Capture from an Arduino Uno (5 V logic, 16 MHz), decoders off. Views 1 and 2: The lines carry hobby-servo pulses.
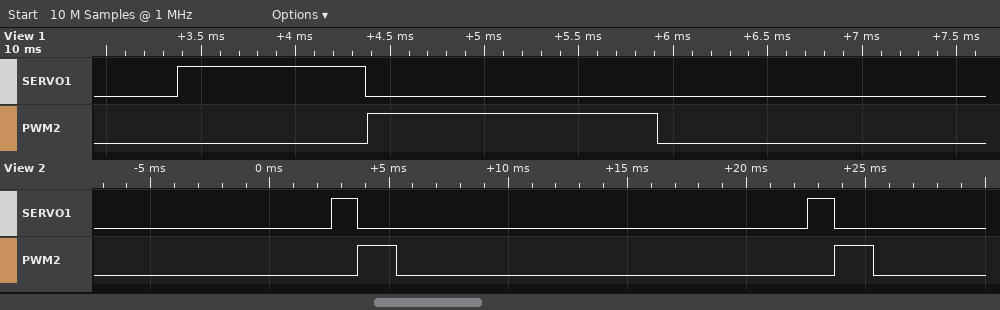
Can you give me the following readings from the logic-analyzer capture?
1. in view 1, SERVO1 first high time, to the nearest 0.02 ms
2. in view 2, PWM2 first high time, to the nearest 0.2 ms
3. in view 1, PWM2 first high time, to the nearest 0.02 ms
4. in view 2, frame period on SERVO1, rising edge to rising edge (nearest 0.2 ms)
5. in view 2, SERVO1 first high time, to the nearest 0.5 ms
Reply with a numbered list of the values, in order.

1. 1.00 ms
2. 1.6 ms
3. 1.54 ms
4. 20.0 ms
5. 1.0 ms
